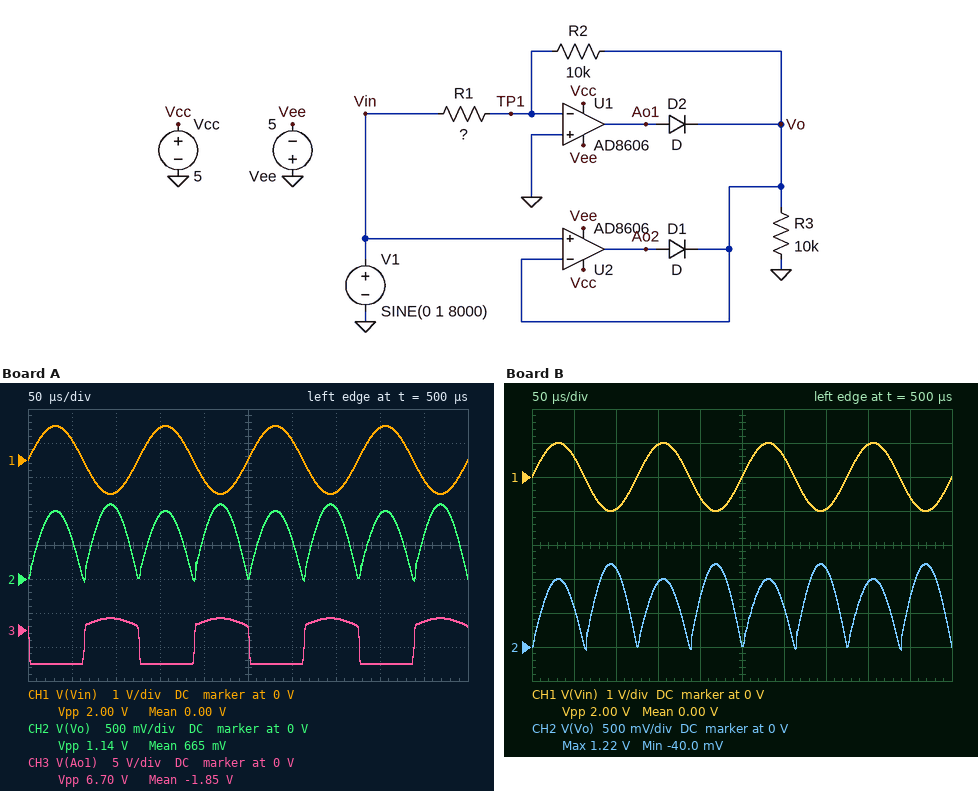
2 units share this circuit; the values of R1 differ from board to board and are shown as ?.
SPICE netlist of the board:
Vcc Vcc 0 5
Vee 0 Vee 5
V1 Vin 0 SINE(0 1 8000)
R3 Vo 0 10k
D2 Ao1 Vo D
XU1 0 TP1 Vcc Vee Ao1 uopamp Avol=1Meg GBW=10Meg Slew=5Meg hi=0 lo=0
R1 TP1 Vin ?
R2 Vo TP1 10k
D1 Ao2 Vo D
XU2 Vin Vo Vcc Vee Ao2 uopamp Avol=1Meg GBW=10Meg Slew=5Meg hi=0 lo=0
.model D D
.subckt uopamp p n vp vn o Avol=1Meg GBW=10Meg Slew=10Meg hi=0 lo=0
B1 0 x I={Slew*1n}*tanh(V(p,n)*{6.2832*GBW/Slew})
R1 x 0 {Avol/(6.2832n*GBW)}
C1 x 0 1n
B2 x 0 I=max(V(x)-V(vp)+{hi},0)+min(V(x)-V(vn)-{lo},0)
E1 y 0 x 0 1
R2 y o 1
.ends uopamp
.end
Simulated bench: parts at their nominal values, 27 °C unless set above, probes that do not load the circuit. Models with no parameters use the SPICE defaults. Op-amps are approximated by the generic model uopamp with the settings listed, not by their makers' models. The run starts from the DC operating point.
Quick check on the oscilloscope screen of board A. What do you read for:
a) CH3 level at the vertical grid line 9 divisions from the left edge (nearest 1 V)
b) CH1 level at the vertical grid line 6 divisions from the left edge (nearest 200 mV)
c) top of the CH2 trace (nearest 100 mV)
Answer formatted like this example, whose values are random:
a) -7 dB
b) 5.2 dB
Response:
a) 1 V
b) 600 mV
c) 1.1 V
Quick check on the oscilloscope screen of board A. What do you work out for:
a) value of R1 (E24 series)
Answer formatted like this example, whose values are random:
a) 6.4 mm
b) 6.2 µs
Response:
a) 9.1 kΩ
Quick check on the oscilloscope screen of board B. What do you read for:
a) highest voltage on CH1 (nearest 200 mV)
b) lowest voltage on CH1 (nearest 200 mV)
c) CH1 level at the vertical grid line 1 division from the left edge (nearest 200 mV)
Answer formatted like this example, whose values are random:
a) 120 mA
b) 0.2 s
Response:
a) 1.0 V
b) -1.0 V
c) 600 mV
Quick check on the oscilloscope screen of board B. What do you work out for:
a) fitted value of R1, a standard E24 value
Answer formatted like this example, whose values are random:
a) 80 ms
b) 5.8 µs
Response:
a) 8.2 kΩ
